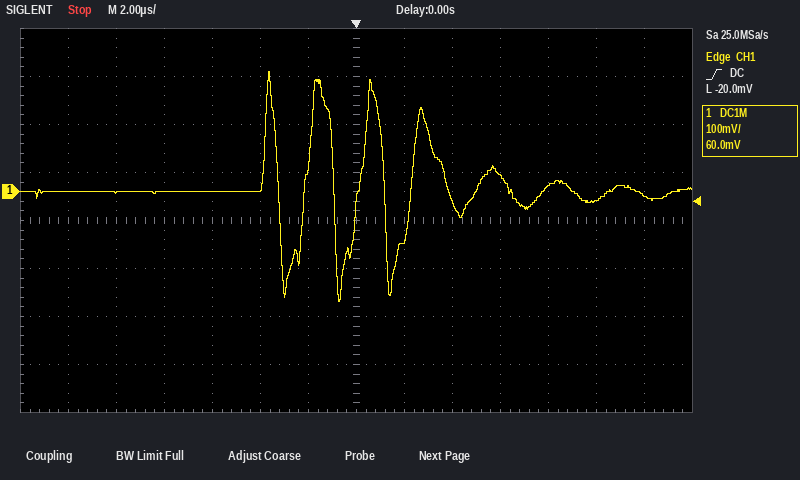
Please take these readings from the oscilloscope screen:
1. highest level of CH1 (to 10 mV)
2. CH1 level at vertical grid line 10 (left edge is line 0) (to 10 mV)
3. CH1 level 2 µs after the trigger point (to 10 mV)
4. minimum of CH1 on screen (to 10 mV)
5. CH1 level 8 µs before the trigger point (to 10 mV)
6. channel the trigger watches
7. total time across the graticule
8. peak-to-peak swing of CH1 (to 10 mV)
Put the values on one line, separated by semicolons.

250 mV; 30 mV; -100 mV; -230 mV; 0 mV; CH1; 28 µs; 480 mV
